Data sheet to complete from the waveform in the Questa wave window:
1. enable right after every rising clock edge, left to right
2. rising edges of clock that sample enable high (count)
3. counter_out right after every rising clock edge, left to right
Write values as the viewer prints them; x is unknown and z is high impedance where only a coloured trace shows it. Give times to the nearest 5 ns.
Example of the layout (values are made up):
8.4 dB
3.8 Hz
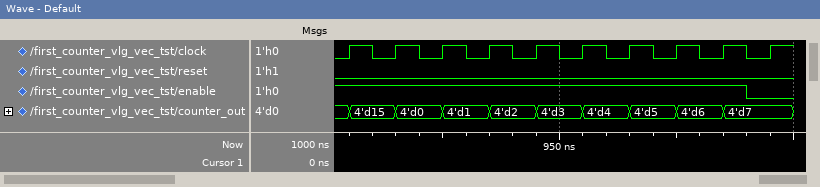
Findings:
1 1 1 1 1 1 1 1 1 0
9
4'd15, 4'd0, 4'd1, 4'd2, 4'd3, 4'd4, 4'd5, 4'd6, 4'd7, 4'd7
